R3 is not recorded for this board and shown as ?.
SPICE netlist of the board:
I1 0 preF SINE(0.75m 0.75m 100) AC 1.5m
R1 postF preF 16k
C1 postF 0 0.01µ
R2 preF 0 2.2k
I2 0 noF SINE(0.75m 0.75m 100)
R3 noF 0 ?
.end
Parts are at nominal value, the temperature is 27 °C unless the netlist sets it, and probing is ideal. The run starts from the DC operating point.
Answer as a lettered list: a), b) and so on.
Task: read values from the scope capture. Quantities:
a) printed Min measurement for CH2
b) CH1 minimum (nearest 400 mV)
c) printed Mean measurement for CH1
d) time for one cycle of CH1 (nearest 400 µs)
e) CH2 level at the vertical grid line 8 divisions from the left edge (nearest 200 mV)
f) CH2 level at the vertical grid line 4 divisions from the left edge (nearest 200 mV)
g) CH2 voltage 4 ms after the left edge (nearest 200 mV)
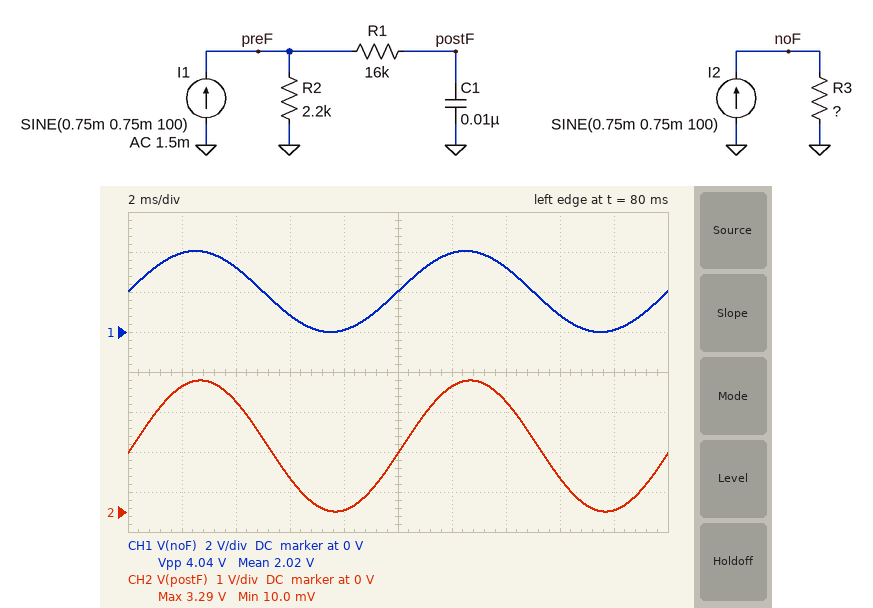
a) 10.0 mV
b) 0 V
c) 2.02 V
d) 10.0 ms
e) 800 mV
f) 0 V
g) 2.8 V
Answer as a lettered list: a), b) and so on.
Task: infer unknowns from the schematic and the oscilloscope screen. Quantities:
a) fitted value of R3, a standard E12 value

a) 2.7 kΩ
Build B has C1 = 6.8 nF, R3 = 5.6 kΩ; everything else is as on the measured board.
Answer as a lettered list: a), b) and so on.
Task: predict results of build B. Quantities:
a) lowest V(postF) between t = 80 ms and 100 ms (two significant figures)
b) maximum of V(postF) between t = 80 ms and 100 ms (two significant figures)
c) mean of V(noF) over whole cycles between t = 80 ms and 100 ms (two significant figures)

a) 5.0 mV
b) 3.3 V
c) 4.2 V
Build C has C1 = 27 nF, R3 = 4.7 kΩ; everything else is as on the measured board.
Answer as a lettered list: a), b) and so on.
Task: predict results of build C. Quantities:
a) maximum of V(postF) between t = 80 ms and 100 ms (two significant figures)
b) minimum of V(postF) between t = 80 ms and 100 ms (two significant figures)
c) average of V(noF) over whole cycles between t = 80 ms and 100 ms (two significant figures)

a) 3.2 V
b) 73 mV
c) 3.5 V
